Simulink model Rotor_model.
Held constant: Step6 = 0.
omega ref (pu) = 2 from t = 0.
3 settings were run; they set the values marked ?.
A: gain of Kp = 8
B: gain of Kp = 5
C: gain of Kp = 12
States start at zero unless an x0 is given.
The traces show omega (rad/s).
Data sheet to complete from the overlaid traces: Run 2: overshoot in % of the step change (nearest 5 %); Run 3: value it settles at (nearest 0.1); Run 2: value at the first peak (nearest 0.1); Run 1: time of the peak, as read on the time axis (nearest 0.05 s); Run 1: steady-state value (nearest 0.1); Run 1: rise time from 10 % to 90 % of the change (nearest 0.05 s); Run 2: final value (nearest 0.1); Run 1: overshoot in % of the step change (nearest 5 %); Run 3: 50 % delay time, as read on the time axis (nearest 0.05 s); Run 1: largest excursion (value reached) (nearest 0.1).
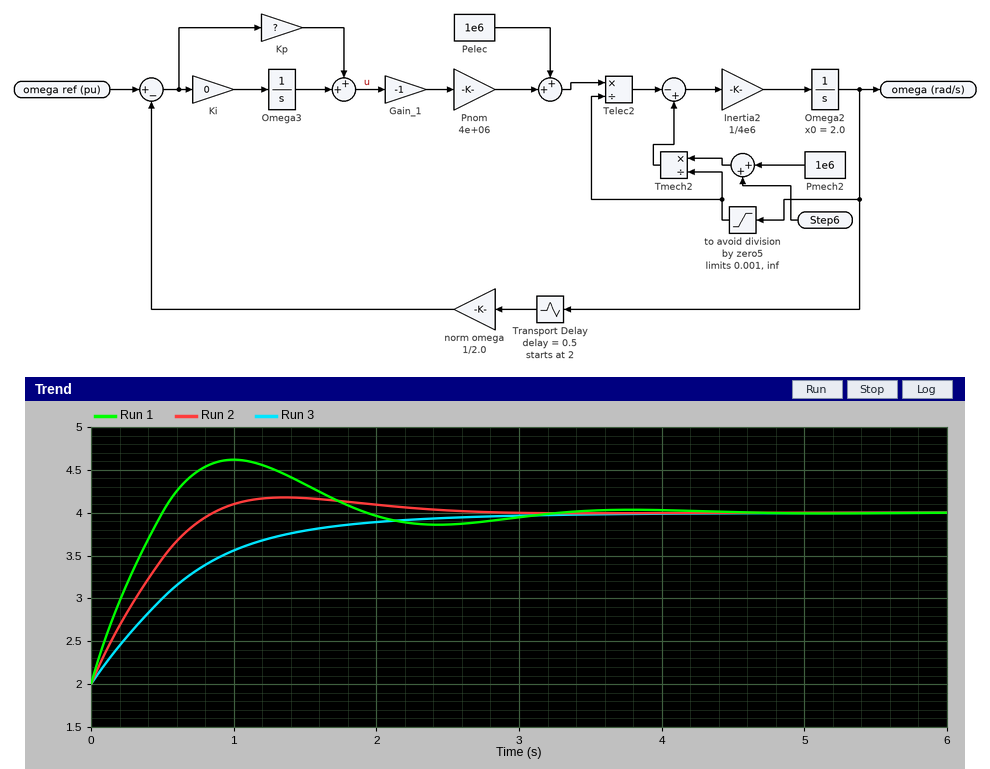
10 %
4.0
4.2
1.00 s
4.0
0.40 s
4.0
30 %
0.50 s
4.6
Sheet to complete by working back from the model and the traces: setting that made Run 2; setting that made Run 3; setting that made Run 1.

A
B
C
